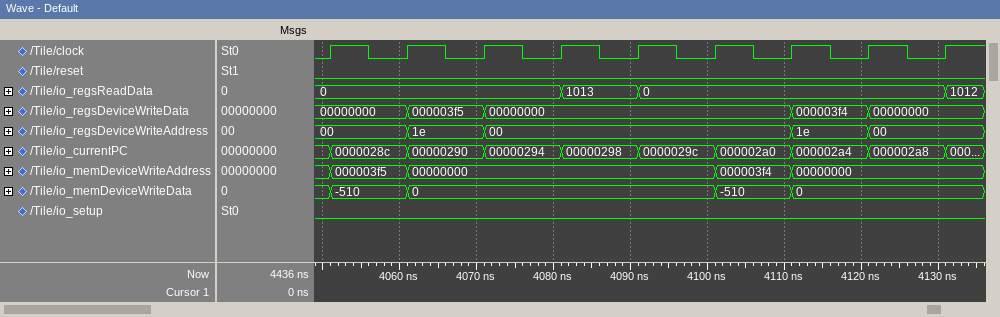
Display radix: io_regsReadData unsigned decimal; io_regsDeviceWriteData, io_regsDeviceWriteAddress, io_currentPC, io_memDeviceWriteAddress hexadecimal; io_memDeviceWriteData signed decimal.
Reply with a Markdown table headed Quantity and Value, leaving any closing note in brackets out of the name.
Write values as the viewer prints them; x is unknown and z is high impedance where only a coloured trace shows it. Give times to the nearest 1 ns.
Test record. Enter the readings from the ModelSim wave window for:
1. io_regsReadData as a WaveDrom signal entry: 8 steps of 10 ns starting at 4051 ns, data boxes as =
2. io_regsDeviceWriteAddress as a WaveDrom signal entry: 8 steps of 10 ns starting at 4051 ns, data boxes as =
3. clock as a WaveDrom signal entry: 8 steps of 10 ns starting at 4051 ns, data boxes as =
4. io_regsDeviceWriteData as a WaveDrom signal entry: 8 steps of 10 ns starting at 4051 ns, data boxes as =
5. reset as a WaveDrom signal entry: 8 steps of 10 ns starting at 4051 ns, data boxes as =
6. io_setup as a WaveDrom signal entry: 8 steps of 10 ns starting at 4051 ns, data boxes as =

| Quantity | Value |
|---|---|
| io_regsReadData as a WaveDrom signal entry: 8 steps of 10 ns starting at 4051 ns, data boxes as = | {name: 'io_regsReadData', wave: '=..==...', data: '0 1013 0'} |
| io_regsDeviceWriteAddress as a WaveDrom signal entry: 8 steps of 10 ns starting at 4051 ns, data boxes as = | {name: 'io_regsDeviceWriteAddress', wave: '===...==', data: '00 1e 00 1e 00'} |
| clock as a WaveDrom signal entry: 8 steps of 10 ns starting at 4051 ns, data boxes as = | {name: 'clock', wave: 'p.......'} |
| io_regsDeviceWriteData as a WaveDrom signal entry: 8 steps of 10 ns starting at 4051 ns, data boxes as = | {name: 'io_regsDeviceWriteData', wave: '===...==', data: '00000000 000003f5 00000000 000003f4 00000000'} |
| reset as a WaveDrom signal entry: 8 steps of 10 ns starting at 4051 ns, data boxes as = | {name: 'reset', wave: '0.......'} |
| io_setup as a WaveDrom signal entry: 8 steps of 10 ns starting at 4051 ns, data boxes as = | {name: 'io_setup', wave: '0.......'} |
